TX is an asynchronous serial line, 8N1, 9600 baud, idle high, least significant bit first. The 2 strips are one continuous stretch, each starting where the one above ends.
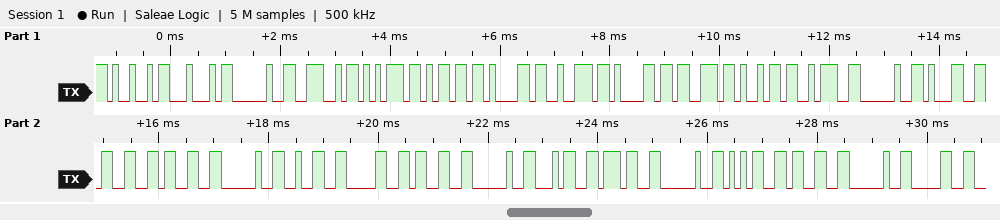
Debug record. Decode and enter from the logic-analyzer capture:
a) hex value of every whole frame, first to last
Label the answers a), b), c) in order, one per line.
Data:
a) 0x49 0x44 0x20 0x4E 0x75 0x6D 0x61 0x72 0x61 0x73 0x69 0x3A 0x20 0x31 0x33 0x33 0x20 0x32 0x30 0x33 0x20 0x34 0x37 0x20 0x35 0x33 0x20 0x30
